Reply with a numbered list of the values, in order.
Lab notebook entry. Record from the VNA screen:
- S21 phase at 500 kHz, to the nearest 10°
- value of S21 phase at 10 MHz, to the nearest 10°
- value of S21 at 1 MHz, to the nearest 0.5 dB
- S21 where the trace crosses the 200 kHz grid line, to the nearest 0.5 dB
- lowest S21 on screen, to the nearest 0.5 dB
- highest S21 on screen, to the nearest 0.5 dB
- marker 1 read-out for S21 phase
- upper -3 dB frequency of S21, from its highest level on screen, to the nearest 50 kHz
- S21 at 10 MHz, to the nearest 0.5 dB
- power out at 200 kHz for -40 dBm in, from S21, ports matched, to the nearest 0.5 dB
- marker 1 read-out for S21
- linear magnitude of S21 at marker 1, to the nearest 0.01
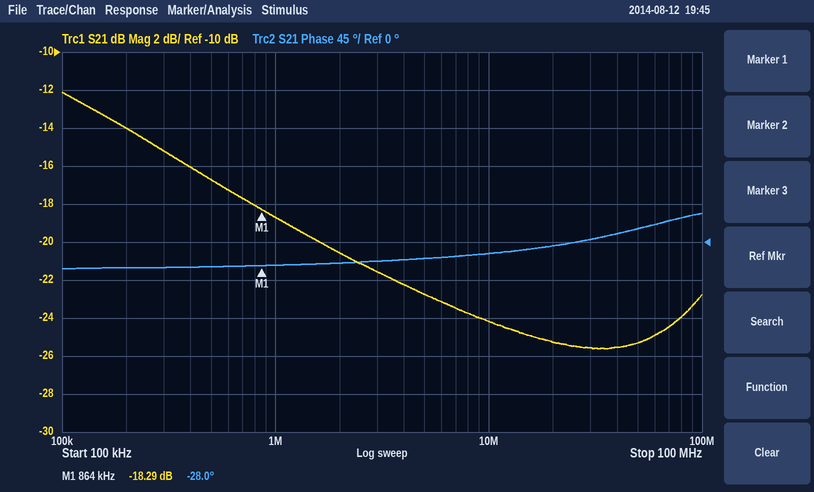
1. -30°
2. -10°
3. -18.5 dB
4. -14.0 dB
5. -25.5 dB
6. -12.0 dB
7. -28.0°
8. 300 kHz
9. -24.0 dB
10. -54.0 dBm
11. -18.29 dB
12. 0.12
